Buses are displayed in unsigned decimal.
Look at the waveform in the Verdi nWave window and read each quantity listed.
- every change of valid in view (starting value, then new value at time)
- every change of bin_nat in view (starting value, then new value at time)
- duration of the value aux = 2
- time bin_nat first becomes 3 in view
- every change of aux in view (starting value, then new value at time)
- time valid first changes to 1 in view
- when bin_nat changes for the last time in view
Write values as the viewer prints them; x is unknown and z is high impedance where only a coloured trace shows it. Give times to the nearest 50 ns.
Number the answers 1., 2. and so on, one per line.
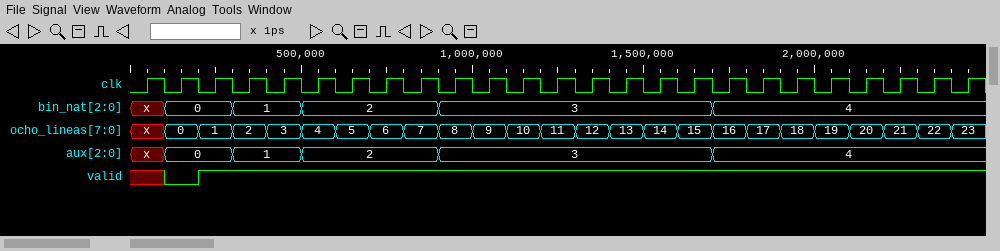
1. x, 0 at 100 ns, 1 at 200 ns
2. x, 0 at 100 ns, 1 at 300 ns, 2 at 500 ns, 3 at 900 ns, 4 at 1700 ns
3. 400 ns
4. 900 ns
5. x, 0 at 100 ns, 1 at 300 ns, 2 at 500 ns, 3 at 900 ns, 4 at 1700 ns
6. 200 ns
7. 1700 ns
